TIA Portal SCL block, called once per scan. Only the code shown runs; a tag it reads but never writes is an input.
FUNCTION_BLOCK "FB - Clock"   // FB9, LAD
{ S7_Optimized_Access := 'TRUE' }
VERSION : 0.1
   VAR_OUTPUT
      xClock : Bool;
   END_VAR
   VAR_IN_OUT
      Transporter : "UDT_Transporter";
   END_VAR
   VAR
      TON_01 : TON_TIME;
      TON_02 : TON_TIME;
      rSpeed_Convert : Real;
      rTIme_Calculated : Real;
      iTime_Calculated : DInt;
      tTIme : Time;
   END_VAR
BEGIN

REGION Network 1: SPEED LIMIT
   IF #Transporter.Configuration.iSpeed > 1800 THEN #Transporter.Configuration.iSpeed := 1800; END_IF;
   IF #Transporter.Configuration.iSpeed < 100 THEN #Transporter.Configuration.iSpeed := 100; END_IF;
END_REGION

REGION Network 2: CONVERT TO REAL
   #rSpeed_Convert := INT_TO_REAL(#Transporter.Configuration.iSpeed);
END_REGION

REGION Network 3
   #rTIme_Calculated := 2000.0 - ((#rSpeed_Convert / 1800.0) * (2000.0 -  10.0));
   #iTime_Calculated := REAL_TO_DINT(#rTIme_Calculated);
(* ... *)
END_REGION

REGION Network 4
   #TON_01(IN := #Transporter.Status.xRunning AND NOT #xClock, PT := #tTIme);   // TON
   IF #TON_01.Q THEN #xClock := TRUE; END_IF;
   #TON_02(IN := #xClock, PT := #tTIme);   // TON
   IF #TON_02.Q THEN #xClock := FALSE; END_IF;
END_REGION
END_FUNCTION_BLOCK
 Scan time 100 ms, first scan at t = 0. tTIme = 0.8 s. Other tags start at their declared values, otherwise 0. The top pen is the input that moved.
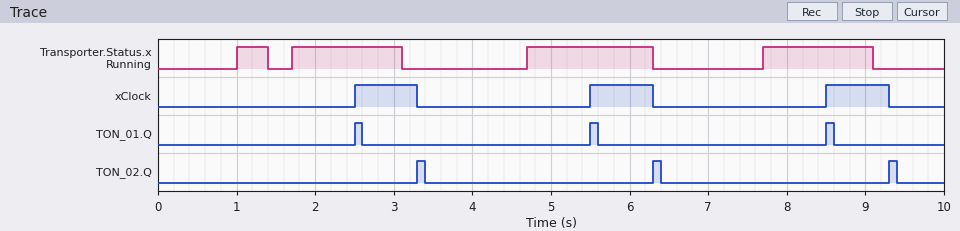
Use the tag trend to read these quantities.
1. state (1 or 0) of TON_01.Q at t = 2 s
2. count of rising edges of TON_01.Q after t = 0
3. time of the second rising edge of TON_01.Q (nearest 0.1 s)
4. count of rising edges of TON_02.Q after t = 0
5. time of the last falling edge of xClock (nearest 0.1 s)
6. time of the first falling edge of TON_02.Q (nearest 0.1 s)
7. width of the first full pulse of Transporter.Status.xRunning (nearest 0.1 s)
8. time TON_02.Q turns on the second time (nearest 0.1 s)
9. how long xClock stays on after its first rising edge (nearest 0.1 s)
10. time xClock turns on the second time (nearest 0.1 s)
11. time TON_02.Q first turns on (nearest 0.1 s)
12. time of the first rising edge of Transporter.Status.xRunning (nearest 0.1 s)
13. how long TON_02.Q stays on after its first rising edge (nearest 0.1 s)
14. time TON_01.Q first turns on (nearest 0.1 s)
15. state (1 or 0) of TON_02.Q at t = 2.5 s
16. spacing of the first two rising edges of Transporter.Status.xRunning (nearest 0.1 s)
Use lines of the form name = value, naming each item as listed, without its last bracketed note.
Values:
state (1 or 0) of TON_01.Q at t = 2 s = 0
count of rising edges of TON_01.Q after t = 0 = 3
time of the second rising edge of TON_01.Q = 5.5 s
count of rising edges of TON_02.Q after t = 0 = 3
time of the last falling edge of xClock = 9.3 s
time of the first falling edge of TON_02.Q = 3.4 s
width of the first full pulse of Transporter.Status.xRunning = 0.4 s
time TON_02.Q turns on the second time = 6.3 s
how long xClock stays on after its first rising edge = 0.8 s
time xClock turns on the second time = 5.5 s
time TON_02.Q first turns on = 3.3 s
time of the first rising edge of Transporter.Status.xRunning = 1.0 s
how long TON_02.Q stays on after its first rising edge = 0.1 s
time TON_01.Q first turns on = 2.5 s
state (1 or 0) of TON_02.Q at t = 2.5 s = 0
spacing of the first two rising edges of Transporter.Status.xRunning = 0.7 s
